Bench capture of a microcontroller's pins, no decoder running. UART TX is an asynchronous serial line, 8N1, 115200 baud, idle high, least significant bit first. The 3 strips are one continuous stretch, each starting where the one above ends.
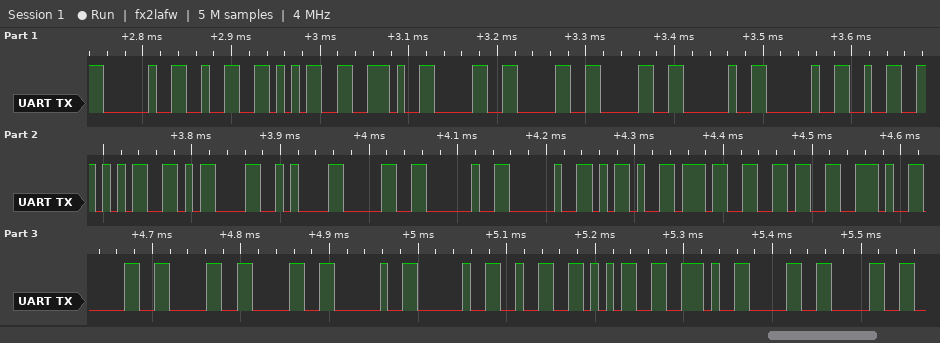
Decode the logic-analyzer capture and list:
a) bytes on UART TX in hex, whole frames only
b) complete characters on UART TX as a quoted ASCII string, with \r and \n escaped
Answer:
20 32 35 2E 30 30 30 20 20 32 35 0D 0A 30 20 20 2D 37 36 2E 30 30 30 20 20 32 35 2E 30 30
" 25.000  25\r\n0  -76.000  25.00"
